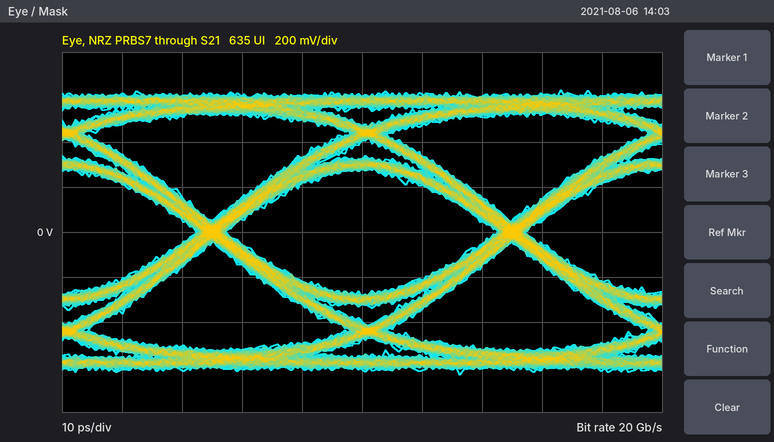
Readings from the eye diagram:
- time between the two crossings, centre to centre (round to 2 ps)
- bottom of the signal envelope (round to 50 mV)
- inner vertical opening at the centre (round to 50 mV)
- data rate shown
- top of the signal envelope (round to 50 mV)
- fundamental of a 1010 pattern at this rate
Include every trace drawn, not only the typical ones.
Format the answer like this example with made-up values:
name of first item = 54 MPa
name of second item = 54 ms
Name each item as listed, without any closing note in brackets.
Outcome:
time between the two crossings, centre to centre = 50 ps
bottom of the signal envelope = -650 mV
inner vertical opening at the centre = 550 mV
data rate shown = 20 Gb/s
top of the signal envelope = 650 mV
fundamental of a 1010 pattern at this rate = 10 GHz
